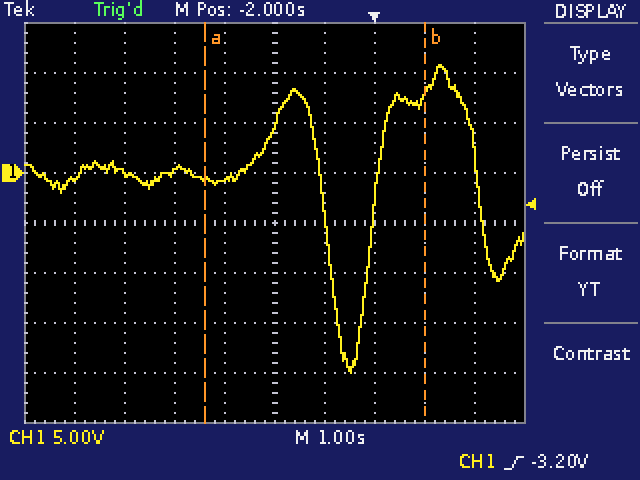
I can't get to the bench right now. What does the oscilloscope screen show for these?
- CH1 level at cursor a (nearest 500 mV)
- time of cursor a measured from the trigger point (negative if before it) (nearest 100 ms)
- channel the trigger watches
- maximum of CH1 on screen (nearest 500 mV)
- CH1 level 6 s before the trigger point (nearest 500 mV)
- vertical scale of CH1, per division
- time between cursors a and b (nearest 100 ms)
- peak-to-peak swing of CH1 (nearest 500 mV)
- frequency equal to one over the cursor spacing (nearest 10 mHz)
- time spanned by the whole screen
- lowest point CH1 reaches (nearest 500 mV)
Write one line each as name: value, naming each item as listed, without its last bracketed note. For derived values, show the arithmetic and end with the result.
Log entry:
CH1 level at cursor a: -500 mV
time of cursor a measured from the trigger point (negative if before it): -3.4 s
channel the trigger watches: CH1
maximum of CH1 on screen: 11.0 V
CH1 level 6 s before the trigger point: -500 mV
vertical scale of CH1, per division: 5 V
time between cursors a and b: 4.4 s
peak-to-peak swing of CH1: 11.0 V − (-20.0 V) = 31.0 V
frequency equal to one over the cursor spacing: 1 / 4.4 s ≈ 230 mHz
time spanned by the whole screen: 10 s
lowest point CH1 reaches: -20.0 V
